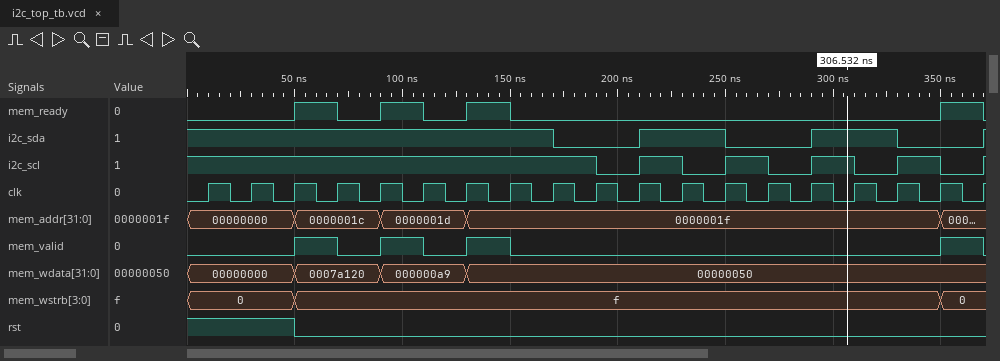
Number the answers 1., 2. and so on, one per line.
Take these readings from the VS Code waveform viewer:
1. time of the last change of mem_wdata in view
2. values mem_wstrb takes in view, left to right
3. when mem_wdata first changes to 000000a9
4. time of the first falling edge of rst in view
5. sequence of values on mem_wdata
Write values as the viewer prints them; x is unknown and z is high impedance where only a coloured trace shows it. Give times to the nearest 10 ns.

1. 130 ns
2. 0, f, 0
3. 90 ns
4. 50 ns
5. 00000000, 0007a120, 000000a9, 00000050
